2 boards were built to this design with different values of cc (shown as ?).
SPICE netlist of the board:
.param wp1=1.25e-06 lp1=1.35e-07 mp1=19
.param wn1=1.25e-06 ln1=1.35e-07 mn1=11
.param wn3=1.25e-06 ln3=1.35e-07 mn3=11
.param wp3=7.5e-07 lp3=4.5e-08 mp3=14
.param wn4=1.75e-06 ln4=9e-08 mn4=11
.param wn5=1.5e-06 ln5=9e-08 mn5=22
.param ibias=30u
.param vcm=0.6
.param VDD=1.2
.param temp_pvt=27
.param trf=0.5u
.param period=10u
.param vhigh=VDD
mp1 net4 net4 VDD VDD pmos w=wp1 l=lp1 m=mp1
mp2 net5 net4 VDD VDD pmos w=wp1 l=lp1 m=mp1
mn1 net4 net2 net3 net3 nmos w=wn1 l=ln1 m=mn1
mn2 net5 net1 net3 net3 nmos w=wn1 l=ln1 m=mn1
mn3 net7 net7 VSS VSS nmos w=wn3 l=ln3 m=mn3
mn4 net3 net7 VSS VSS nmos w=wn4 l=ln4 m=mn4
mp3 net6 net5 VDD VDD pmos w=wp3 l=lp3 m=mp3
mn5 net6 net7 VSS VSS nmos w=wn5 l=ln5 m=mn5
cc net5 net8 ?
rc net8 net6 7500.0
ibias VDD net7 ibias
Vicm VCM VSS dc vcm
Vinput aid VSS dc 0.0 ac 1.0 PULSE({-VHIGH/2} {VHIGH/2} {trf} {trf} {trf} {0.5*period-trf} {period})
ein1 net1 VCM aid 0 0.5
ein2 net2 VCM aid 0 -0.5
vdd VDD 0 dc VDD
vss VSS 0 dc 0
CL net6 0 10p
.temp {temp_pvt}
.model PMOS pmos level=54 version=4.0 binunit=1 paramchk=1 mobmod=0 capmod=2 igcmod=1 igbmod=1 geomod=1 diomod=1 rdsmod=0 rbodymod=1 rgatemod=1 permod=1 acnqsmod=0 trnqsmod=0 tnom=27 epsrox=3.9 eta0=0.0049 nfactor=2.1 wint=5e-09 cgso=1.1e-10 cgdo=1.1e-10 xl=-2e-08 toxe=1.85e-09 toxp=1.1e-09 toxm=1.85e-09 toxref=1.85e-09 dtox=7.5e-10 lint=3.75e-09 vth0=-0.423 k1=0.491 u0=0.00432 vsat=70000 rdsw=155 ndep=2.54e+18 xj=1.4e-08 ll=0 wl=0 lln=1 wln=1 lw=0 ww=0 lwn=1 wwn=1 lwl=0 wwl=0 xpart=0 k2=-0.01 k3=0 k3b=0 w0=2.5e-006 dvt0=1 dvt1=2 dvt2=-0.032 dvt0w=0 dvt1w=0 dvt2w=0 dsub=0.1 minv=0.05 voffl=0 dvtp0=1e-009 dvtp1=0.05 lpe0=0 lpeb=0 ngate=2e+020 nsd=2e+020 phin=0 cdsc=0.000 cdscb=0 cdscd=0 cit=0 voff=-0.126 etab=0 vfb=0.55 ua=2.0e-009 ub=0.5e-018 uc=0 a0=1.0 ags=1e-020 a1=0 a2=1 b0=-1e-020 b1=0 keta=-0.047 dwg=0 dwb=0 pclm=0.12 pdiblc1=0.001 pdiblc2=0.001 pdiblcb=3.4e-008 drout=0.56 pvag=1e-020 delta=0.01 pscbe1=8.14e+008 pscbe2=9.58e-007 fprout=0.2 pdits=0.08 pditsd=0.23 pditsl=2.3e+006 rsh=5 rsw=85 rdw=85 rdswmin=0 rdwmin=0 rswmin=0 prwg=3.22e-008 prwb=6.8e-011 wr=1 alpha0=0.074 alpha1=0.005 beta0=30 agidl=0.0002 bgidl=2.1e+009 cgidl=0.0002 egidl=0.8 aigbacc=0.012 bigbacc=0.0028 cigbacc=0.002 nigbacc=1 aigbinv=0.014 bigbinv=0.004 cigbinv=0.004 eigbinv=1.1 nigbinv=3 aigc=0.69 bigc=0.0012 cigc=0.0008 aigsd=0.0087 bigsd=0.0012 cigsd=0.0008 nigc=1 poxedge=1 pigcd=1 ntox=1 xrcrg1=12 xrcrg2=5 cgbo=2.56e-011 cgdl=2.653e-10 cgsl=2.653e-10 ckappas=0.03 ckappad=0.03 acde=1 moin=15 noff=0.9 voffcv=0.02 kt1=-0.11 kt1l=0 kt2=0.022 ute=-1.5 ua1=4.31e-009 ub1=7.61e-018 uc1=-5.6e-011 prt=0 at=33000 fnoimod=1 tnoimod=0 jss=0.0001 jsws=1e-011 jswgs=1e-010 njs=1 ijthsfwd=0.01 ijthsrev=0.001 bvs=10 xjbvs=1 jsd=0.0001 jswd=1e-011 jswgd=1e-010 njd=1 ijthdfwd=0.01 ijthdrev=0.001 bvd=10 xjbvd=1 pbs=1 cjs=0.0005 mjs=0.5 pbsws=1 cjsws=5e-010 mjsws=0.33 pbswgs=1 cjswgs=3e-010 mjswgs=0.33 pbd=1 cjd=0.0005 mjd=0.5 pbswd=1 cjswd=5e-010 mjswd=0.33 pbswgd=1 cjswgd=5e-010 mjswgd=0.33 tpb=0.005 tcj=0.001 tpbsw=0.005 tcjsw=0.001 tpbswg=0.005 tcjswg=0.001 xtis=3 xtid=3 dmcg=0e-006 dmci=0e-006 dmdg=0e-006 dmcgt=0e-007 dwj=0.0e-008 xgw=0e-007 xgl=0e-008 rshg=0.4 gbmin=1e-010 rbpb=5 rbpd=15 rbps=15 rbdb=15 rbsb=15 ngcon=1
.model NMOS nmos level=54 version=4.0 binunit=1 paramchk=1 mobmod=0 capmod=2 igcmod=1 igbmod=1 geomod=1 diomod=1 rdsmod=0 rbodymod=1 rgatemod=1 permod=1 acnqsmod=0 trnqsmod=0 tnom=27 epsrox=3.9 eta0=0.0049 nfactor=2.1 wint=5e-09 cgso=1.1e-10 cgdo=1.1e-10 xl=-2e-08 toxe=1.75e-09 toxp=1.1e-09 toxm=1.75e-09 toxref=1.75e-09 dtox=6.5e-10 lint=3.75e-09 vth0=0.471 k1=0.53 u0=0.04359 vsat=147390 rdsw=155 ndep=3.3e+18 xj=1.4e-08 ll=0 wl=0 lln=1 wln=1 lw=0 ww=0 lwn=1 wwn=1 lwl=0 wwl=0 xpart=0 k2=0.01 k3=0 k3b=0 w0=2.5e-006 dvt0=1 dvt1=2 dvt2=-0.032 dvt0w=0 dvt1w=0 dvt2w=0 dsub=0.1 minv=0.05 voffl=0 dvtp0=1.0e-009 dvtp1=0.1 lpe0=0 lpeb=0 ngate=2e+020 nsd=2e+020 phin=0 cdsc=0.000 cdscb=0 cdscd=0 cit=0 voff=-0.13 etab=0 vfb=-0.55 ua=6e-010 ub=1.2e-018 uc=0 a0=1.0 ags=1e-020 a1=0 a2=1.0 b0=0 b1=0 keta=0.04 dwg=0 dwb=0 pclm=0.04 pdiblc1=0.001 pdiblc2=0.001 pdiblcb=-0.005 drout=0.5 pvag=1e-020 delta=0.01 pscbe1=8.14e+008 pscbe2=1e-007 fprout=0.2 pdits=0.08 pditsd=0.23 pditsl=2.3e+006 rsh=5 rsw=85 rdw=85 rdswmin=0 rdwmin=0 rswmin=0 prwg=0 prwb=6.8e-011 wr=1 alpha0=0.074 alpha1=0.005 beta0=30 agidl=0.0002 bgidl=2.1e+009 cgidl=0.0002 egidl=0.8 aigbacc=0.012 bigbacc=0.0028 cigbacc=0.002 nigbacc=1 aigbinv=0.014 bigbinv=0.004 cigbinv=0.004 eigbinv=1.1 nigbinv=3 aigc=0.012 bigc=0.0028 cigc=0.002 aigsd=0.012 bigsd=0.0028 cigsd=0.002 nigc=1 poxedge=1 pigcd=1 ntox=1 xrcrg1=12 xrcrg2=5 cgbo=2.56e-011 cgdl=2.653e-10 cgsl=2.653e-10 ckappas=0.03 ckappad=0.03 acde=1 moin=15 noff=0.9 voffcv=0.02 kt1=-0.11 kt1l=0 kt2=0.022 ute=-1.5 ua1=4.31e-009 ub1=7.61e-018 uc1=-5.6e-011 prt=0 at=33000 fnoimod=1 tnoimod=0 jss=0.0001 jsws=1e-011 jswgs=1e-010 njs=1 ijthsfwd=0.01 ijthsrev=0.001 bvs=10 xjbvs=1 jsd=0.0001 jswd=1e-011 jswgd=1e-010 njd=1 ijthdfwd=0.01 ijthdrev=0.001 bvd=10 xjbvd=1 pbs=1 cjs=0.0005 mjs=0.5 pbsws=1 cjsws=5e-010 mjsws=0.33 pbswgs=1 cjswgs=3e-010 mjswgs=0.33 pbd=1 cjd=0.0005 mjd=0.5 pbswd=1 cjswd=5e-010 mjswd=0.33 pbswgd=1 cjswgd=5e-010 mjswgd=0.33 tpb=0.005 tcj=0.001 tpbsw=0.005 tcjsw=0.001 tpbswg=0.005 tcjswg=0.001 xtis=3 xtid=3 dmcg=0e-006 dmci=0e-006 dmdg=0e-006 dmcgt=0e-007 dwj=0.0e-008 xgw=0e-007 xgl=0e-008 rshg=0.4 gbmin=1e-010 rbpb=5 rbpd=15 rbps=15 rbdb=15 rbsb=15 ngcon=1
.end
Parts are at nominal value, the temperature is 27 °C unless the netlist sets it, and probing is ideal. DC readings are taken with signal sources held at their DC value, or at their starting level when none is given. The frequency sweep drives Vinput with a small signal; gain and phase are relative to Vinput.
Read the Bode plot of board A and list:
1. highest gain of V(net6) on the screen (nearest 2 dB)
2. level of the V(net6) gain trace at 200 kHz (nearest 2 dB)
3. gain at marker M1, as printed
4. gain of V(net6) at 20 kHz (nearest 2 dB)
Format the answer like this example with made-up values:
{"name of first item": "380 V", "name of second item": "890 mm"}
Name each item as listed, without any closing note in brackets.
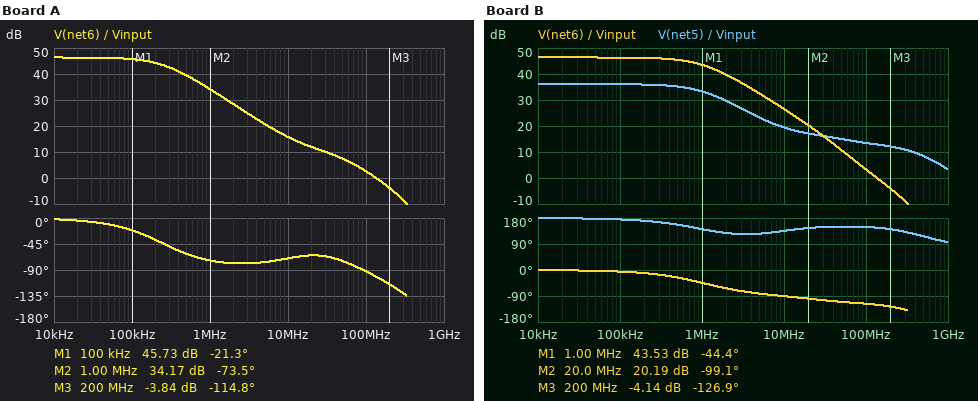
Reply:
{"highest gain of V(net6) on the screen": "46 dB", "level of the V(net6) gain trace at 200 kHz": "44 dB", "gain at marker M1, as printed": "45.73 dB", "gain of V(net6) at 20 kHz": "46 dB"}
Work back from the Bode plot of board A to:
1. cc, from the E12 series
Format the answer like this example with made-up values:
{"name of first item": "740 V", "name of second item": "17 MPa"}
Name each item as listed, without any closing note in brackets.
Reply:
{"cc, from the E12 series": "1.5 pF"}
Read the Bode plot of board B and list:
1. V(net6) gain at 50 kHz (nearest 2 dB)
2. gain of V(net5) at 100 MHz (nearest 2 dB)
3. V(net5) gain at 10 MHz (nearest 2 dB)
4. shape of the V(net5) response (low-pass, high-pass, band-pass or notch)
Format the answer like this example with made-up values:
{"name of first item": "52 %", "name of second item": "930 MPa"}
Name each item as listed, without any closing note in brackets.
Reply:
{"V(net6) gain at 50 kHz": "46 dB", "gain of V(net5) at 100 MHz": "14 dB", "V(net5) gain at 10 MHz": "20 dB", "shape of the V(net5) response": "low-pass"}
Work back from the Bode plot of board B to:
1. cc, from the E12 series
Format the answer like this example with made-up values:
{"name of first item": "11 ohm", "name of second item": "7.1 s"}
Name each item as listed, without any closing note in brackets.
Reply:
{"cc, from the E12 series": "330 fF"}
